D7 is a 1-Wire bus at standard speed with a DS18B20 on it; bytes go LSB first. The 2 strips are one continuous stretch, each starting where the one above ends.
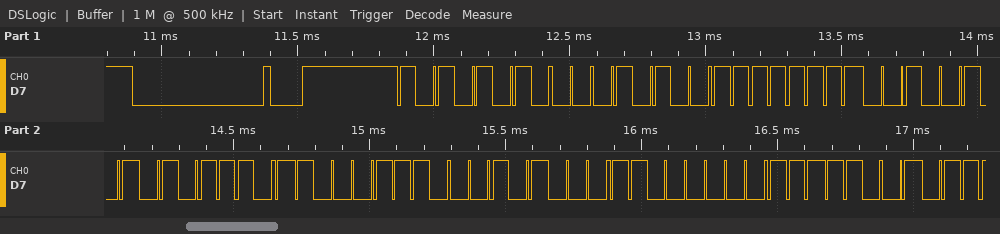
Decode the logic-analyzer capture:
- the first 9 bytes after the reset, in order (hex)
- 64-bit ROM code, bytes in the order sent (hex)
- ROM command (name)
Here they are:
55 28 FF A4 BA 71 14 03 9F
28 FF A4 BA 71 14 03 9F
Match ROM
